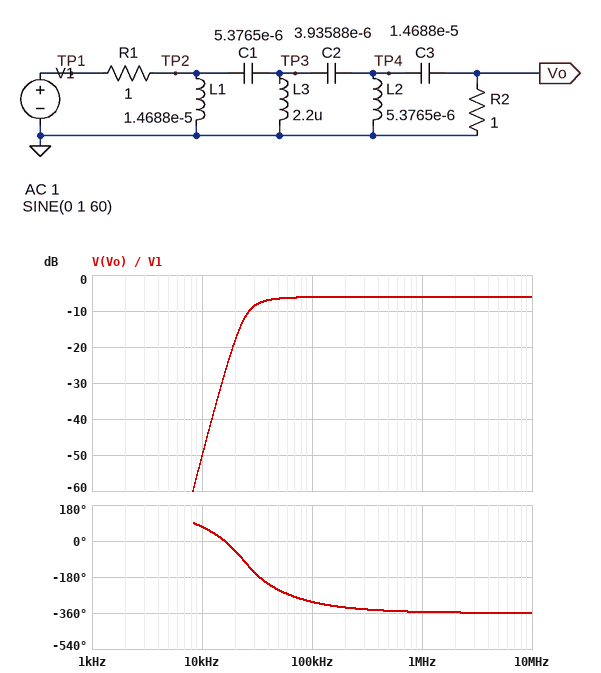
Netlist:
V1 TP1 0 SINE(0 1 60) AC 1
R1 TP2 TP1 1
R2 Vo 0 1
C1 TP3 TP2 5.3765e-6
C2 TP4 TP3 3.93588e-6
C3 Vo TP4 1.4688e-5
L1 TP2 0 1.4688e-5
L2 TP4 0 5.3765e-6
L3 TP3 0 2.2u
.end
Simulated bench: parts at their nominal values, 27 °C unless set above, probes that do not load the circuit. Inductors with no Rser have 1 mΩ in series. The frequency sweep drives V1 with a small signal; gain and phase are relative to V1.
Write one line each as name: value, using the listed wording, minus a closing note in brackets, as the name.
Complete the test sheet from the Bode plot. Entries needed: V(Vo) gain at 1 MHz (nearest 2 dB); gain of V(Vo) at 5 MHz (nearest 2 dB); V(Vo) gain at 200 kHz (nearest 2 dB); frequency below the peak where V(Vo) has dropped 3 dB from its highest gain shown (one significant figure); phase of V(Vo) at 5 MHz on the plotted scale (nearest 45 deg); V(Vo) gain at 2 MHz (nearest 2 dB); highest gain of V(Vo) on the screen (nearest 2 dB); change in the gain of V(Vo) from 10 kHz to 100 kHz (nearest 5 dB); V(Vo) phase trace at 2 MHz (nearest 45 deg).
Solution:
V(Vo) gain at 1 MHz: -6 dB
gain of V(Vo) at 5 MHz: -6 dB
V(Vo) gain at 200 kHz: -6 dB
frequency below the peak where V(Vo) has dropped 3 dB from its highest gain shown: 30 kHz
phase of V(Vo) at 5 MHz on the plotted scale: -360 deg
V(Vo) gain at 2 MHz: -6 dB
highest gain of V(Vo) on the screen: -6 dB
change in the gain of V(Vo) from 10 kHz to 100 kHz: 45 dB
V(Vo) phase trace at 2 MHz: -360 deg
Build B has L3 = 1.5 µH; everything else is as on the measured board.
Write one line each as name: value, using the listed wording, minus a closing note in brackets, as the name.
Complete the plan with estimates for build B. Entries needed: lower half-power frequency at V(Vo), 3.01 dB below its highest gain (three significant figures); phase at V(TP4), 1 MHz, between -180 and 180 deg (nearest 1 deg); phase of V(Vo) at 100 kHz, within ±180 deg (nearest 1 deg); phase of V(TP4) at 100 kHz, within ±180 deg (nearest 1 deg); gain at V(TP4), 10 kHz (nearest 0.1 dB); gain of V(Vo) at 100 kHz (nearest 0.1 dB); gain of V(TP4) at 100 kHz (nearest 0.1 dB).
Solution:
lower half-power frequency at V(Vo), 3.01 dB below its highest gain: 40.2 kHz
phase at V(TP4), 1 MHz, between -180 and 180 deg: 6 deg
phase of V(Vo) at 100 kHz, within ±180 deg: 65 deg
phase of V(TP4) at 100 kHz, within ±180 deg: 59 deg
gain at V(TP4), 10 kHz: -50.5 dB
gain of V(Vo) at 100 kHz: -6.5 dB
gain of V(TP4) at 100 kHz: -6.4 dB
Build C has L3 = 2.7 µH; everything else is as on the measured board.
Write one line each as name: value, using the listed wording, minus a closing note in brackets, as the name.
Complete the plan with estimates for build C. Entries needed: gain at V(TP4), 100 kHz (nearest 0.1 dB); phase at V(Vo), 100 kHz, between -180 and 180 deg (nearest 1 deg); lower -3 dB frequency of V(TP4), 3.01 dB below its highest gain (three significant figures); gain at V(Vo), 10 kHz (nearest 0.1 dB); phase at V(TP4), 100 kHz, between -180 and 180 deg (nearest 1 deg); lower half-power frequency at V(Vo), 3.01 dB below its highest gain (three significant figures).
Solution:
gain at V(TP4), 100 kHz: -6.0 dB
phase at V(Vo), 100 kHz, between -180 and 180 deg: 52 deg
lower -3 dB frequency of V(TP4), 3.01 dB below its highest gain: 24.2 kHz
gain at V(Vo), 10 kHz: -48.3 dB
phase at V(TP4), 100 kHz, between -180 and 180 deg: 46 deg
lower half-power frequency at V(Vo), 3.01 dB below its highest gain: 25.3 kHz
